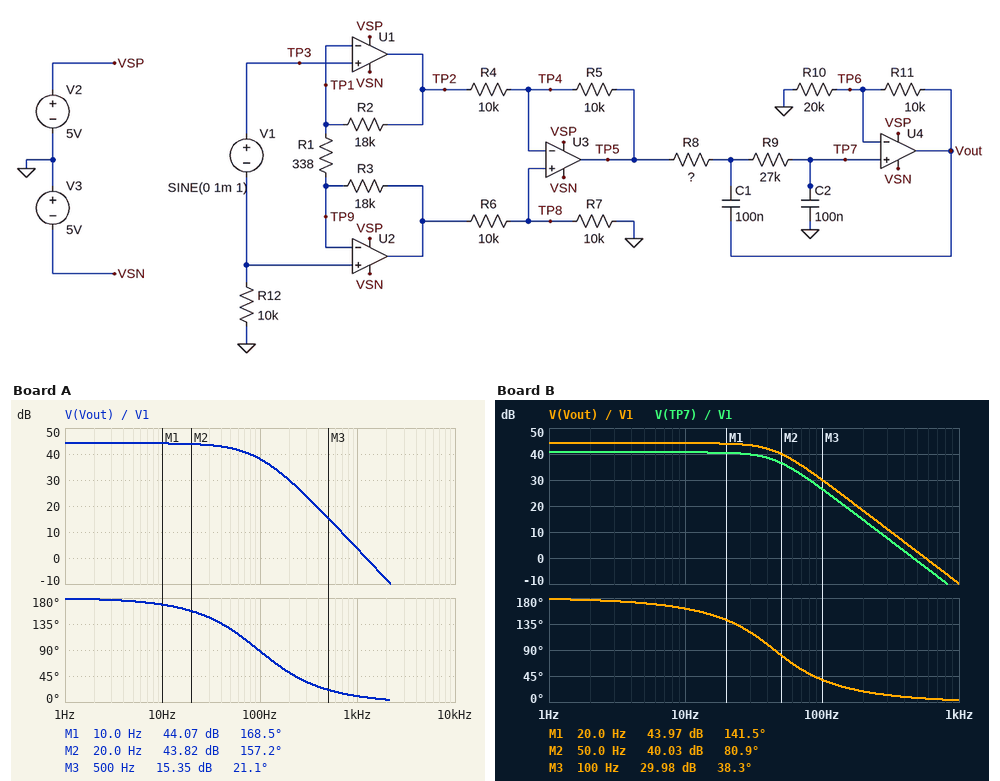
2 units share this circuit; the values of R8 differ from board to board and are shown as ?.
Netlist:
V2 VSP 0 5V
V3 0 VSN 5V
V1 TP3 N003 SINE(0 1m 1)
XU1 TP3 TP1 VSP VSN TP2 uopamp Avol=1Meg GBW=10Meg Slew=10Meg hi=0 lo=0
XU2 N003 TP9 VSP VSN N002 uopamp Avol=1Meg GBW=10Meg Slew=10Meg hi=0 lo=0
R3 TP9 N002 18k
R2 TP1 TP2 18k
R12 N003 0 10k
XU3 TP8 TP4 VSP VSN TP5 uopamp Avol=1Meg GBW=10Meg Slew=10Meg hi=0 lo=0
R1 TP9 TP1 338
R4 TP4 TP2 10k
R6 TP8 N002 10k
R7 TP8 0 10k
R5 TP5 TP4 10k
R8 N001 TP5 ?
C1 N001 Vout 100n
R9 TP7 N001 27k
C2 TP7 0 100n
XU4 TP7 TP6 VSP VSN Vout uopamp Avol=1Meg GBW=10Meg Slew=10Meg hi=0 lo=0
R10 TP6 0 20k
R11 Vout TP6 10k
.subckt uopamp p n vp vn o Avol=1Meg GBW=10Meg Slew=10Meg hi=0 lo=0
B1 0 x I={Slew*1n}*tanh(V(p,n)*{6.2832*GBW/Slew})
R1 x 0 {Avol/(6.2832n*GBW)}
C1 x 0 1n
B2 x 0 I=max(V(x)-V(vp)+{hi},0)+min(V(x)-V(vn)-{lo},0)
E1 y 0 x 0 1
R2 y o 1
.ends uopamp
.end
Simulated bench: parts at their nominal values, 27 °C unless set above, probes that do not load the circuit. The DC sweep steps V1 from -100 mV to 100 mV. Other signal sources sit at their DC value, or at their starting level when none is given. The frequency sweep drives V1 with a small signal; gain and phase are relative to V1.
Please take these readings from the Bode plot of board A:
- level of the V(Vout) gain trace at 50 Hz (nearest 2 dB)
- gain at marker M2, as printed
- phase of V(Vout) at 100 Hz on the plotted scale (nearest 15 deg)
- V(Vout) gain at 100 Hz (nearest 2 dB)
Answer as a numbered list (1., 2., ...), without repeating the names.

1. 42 dB
2. 43.82 dB
3. 90 deg
4. 38 dB
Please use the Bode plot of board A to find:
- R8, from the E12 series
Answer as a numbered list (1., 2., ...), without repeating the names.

1. 10 kΩ
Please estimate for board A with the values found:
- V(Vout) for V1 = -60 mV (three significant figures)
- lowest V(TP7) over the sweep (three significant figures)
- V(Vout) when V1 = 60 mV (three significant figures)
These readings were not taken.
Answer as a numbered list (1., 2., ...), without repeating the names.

1. 5.01 V
2. -5.01 V
3. -5.01 V
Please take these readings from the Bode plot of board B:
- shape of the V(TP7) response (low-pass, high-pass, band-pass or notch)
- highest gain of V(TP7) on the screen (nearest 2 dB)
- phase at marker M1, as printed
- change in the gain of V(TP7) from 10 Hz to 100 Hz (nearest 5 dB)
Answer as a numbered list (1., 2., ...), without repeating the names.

1. low-pass
2. 40 dB
3. 141.5 deg
4. -15 dB
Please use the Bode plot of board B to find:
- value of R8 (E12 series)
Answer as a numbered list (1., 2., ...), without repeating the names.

1. 47 kΩ
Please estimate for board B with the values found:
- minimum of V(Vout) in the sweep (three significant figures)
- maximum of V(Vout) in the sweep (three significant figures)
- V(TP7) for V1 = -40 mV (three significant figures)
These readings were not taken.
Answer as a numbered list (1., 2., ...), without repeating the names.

1. -5.01 V
2. 5.01 V
3. 4.30 V
